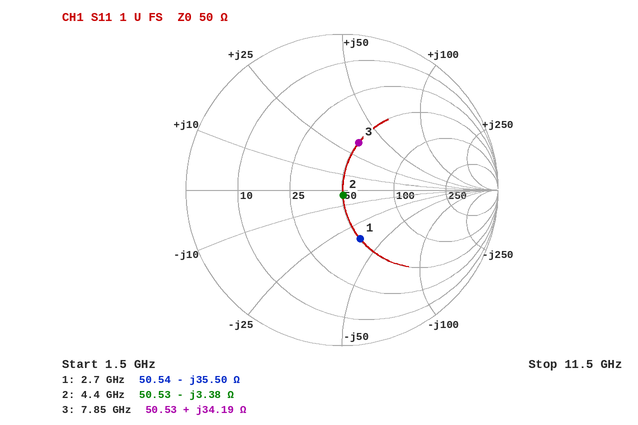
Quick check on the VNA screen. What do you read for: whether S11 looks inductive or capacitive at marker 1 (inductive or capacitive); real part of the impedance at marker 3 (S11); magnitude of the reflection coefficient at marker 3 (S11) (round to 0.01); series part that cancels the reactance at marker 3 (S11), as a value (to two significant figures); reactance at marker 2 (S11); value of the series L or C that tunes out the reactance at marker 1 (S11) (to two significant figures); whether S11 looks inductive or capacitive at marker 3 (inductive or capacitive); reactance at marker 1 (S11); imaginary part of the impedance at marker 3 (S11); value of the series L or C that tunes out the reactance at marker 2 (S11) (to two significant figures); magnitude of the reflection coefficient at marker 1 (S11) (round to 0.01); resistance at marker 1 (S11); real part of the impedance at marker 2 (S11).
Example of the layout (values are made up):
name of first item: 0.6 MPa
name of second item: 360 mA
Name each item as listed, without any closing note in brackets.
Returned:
whether S11 looks inductive or capacitive at marker 1: capacitive
real part of the impedance at marker 3: 50.53 Ω
magnitude of the reflection coefficient at marker 3 (S11): 0.32
series part that cancels the reactance at marker 3 (S11), as a value: 590 fF
reactance at marker 2: -3.38 Ω
value of the series L or C that tunes out the reactance at marker 1 (S11): 2.1 nH
whether S11 looks inductive or capacitive at marker 3: inductive
reactance at marker 1: -35.50 Ω
imaginary part of the impedance at marker 3: +34.19 Ω
value of the series L or C that tunes out the reactance at marker 2 (S11): 120 pH
magnitude of the reflection coefficient at marker 1 (S11): 0.33
resistance at marker 1: 50.54 Ω
real part of the impedance at marker 2: 50.53 Ω
